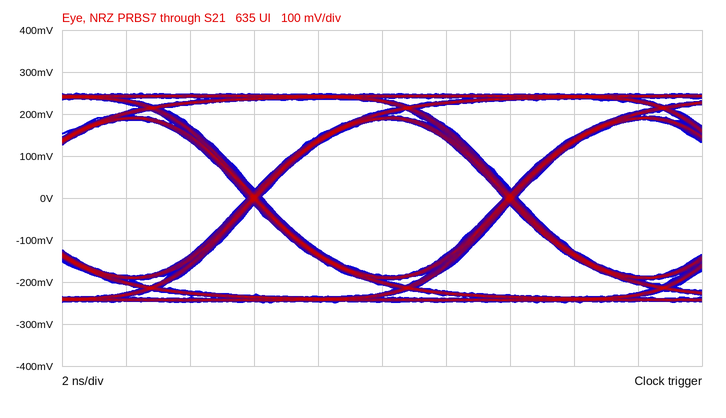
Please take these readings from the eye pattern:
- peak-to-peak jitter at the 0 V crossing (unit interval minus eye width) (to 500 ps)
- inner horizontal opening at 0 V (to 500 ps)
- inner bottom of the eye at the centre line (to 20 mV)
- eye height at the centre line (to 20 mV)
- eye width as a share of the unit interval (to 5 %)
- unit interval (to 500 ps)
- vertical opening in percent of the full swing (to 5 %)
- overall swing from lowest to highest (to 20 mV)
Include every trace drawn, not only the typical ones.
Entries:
500 ps
7.5 ns
-180 mV
380 mV
95 %
8.0 ns
75 %
500 mV
